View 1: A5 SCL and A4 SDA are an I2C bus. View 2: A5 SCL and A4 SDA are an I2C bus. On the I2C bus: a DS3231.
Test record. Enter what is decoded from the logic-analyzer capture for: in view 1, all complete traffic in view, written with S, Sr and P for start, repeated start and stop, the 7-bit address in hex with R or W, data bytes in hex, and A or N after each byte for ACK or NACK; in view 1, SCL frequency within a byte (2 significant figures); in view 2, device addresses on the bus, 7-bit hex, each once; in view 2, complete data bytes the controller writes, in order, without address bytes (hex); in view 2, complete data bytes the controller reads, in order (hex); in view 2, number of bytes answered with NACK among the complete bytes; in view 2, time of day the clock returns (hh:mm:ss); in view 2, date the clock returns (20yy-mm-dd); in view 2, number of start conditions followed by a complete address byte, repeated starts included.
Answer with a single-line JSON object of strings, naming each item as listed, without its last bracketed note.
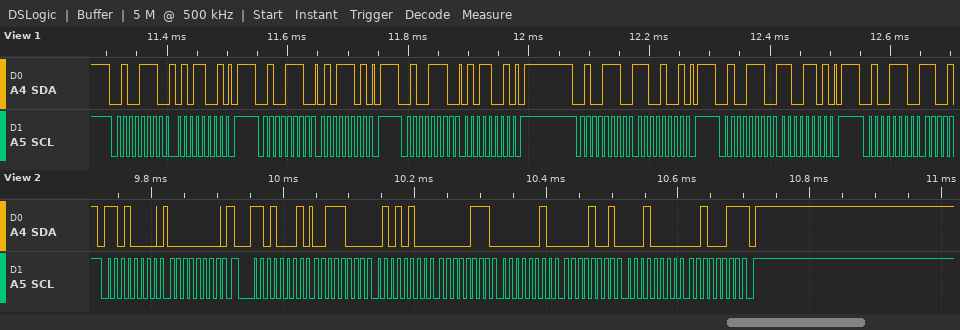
{"in view 1, all complete traffic in view, written with S, Sr and P for start, repeated start and stop, the 7-bit address in hex with R or W, data bytes in hex, and A or N after each byte for ACK or NACK": "S 27W A 59 A P S 27W A 5D A P S 27W A 59 A P S 27W A C9 A P S 27W A CD A P S 27W A", "in view 1, SCL frequency within a byte": "100 kHz", "in view 2, device addresses on the bus, 7-bit hex, each once": "0x68", "in view 2, complete data bytes the controller writes, in order, without address bytes": "00", "in view 2, complete data bytes the controller reads, in order": "38 54 07 02 09 10 23", "in view 2, number of bytes answered with NACK among the complete bytes": "1", "in view 2, time of day the clock returns": "07:54:38", "in view 2, date the clock returns": "2023-10-09", "in view 2, number of start conditions followed by a complete address byte, repeated starts included": "2"}
